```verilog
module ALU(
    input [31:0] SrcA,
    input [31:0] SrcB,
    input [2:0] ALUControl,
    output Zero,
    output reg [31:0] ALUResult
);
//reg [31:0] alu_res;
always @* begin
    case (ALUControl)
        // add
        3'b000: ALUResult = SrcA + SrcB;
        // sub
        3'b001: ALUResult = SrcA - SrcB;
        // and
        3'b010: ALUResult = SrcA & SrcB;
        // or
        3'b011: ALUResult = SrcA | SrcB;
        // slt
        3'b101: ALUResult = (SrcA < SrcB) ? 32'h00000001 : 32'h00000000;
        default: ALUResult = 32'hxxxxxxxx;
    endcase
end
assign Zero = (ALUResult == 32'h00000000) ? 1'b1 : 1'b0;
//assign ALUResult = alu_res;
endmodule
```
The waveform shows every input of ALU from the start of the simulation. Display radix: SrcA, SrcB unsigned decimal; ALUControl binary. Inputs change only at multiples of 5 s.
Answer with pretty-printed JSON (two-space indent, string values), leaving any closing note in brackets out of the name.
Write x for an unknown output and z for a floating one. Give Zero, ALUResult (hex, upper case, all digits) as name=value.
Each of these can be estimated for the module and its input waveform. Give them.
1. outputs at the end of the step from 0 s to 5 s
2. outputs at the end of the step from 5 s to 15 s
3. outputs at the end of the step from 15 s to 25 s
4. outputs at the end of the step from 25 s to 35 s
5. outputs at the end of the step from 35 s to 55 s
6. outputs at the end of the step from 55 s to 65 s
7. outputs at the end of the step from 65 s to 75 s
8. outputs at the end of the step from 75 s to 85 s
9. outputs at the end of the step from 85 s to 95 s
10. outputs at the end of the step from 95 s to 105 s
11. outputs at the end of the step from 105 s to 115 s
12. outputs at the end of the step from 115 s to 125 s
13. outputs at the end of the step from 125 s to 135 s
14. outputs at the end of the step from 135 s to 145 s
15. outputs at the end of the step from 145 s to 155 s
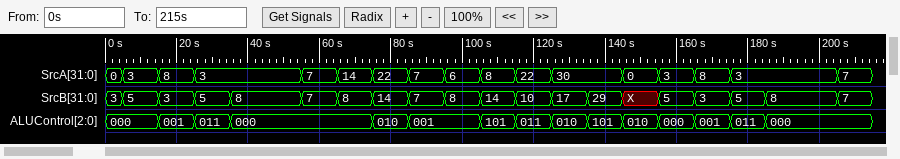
{
  "outputs at the end of the step from 0 s to 5 s": "Zero=0, ALUResult=00000003",
  "outputs at the end of the step from 5 s to 15 s": "Zero=0, ALUResult=00000008",
  "outputs at the end of the step from 15 s to 25 s": "Zero=0, ALUResult=00000005",
  "outputs at the end of the step from 25 s to 35 s": "Zero=0, ALUResult=00000007",
  "outputs at the end of the step from 35 s to 55 s": "Zero=0, ALUResult=0000000B",
  "outputs at the end of the step from 55 s to 65 s": "Zero=0, ALUResult=0000000E",
  "outputs at the end of the step from 65 s to 75 s": "Zero=0, ALUResult=00000016",
  "outputs at the end of the step from 75 s to 85 s": "Zero=0, ALUResult=00000006",
  "outputs at the end of the step from 85 s to 95 s": "Zero=1, ALUResult=00000000",
  "outputs at the end of the step from 95 s to 105 s": "Zero=0, ALUResult=FFFFFFFE",
  "outputs at the end of the step from 105 s to 115 s": "Zero=0, ALUResult=00000001",
  "outputs at the end of the step from 115 s to 125 s": "Zero=0, ALUResult=0000001E",
  "outputs at the end of the step from 125 s to 135 s": "Zero=0, ALUResult=00000010",
  "outputs at the end of the step from 135 s to 145 s": "Zero=1, ALUResult=00000000",
  "outputs at the end of the step from 145 s to 155 s": "Zero=1, ALUResult=00000000"
}
